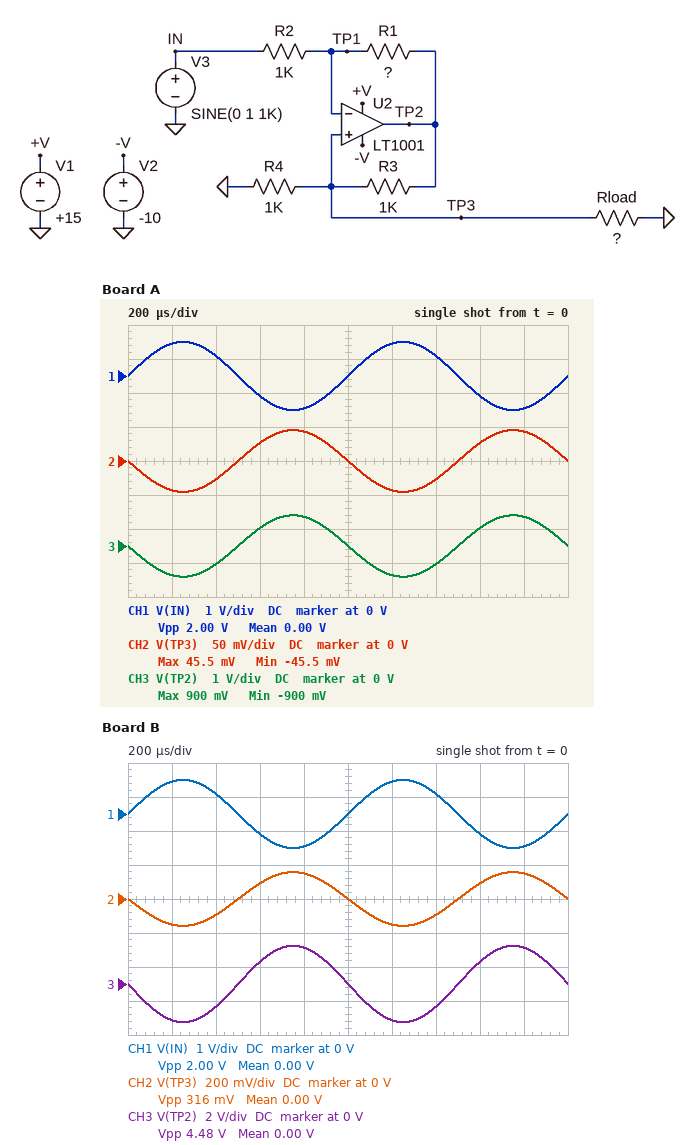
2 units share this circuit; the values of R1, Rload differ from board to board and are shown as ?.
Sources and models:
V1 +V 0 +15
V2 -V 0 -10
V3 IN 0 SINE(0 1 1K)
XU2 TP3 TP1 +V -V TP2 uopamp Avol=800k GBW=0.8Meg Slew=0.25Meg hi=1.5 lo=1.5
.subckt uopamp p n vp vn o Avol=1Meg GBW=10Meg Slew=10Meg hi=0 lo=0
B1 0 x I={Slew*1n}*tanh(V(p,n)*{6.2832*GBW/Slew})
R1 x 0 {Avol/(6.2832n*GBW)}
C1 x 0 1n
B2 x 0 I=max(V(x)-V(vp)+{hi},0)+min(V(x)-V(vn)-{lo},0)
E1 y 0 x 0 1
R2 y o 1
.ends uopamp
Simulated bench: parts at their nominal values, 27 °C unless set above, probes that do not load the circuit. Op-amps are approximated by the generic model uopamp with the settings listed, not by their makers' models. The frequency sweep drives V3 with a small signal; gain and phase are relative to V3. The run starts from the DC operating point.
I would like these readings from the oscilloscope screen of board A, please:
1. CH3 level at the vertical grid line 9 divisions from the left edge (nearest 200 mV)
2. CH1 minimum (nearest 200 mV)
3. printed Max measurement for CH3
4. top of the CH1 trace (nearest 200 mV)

800 mV
-1.0 V
900 mV
1.0 V
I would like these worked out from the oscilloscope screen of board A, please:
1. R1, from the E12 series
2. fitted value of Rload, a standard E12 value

820 Ω
56 Ω
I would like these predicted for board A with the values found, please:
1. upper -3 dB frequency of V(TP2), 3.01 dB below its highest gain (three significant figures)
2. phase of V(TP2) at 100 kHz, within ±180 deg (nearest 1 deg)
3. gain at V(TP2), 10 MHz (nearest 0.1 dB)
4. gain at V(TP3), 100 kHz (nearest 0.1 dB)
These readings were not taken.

399 kHz
166 deg
-28.9 dB
-27.1 dB
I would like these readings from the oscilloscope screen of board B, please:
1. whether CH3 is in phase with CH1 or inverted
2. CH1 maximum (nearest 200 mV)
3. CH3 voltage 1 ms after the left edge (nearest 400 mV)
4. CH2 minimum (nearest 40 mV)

inverted
1.0 V
0 V
-160 mV
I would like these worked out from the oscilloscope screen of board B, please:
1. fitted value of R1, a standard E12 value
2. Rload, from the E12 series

1.8 kΩ
82 Ω
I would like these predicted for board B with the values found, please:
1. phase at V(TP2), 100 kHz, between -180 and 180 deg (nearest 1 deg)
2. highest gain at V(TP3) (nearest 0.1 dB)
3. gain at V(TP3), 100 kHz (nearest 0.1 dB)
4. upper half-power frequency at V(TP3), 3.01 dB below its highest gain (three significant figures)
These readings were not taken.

156 deg
-16.0 dB
-16.8 dB
229 kHz
